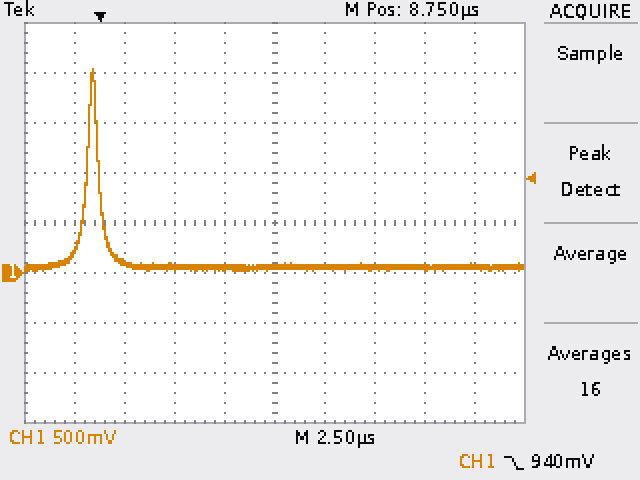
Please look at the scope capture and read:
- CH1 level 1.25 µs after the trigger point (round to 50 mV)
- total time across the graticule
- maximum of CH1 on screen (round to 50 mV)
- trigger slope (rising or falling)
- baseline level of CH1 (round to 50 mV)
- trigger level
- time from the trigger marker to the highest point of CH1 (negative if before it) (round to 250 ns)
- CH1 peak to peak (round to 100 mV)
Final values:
100 mV
25 µs
2.05 V
falling
50 mV
940 mV
-250 ns
2.00 V
